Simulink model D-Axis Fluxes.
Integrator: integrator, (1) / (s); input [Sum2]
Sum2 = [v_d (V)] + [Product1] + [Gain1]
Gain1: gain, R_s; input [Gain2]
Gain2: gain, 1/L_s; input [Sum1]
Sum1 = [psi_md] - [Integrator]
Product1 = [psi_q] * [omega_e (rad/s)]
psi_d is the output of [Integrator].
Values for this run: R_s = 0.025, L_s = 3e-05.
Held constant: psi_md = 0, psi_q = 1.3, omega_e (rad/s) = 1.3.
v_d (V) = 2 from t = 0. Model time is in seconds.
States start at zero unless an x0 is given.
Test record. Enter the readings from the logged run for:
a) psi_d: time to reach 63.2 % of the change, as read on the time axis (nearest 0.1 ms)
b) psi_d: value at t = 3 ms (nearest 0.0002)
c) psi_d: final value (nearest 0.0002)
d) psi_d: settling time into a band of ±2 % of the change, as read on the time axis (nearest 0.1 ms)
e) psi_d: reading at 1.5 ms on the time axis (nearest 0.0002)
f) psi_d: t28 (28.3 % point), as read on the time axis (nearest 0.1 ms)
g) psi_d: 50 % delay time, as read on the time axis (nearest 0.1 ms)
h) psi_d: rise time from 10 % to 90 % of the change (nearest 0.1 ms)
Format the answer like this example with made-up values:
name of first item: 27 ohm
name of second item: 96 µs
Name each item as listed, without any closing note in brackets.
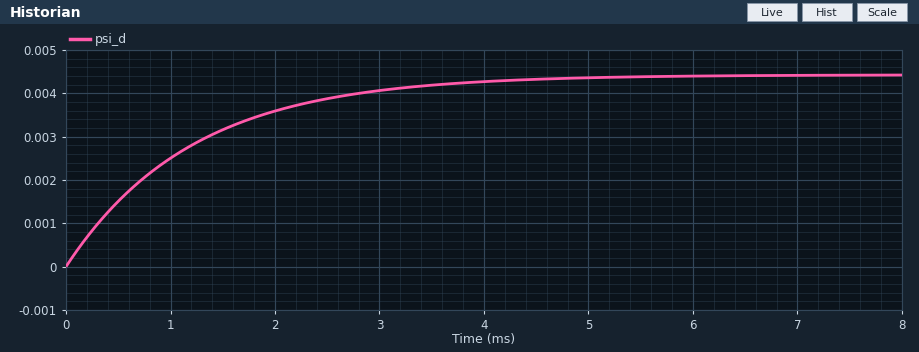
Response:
psi_d: time to reach 63.2 % of the change, as read on the time axis: 1.2 ms
psi_d: value at t = 3 ms: 0.0040
psi_d: final value: 0.0044
psi_d: settling time into a band of ±2 % of the change, as read on the time axis: 4.7 ms
psi_d: reading at 1.5 ms on the time axis: 0.0032
psi_d: t28 (28.3 % point), as read on the time axis: 0.4 ms
psi_d: 50 % delay time, as read on the time axis: 0.8 ms
psi_d: rise time from 10 % to 90 % of the change: 2.6 ms
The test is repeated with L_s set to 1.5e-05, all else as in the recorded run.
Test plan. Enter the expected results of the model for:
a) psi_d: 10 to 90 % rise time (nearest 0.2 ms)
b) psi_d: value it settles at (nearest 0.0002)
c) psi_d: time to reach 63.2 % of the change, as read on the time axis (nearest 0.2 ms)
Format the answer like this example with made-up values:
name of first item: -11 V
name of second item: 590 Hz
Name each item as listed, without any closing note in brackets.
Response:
psi_d: 10 to 90 % rise time: 1.4 ms
psi_d: value it settles at: 0.0022
psi_d: time to reach 63.2 % of the change, as read on the time axis: 0.6 ms
